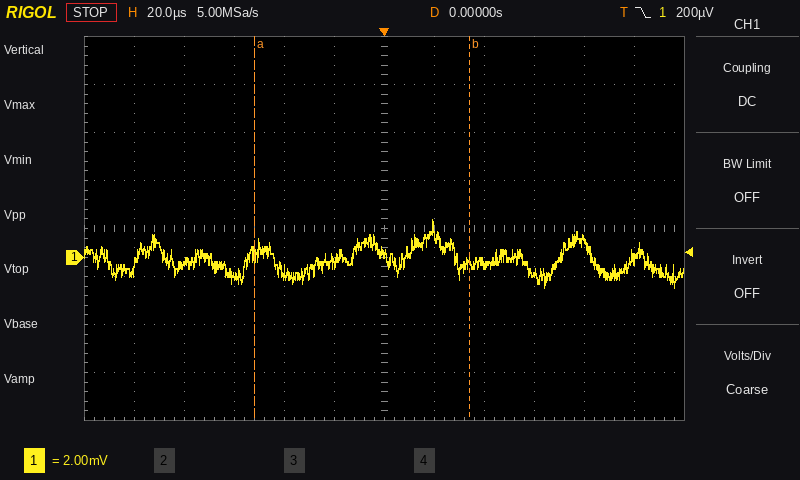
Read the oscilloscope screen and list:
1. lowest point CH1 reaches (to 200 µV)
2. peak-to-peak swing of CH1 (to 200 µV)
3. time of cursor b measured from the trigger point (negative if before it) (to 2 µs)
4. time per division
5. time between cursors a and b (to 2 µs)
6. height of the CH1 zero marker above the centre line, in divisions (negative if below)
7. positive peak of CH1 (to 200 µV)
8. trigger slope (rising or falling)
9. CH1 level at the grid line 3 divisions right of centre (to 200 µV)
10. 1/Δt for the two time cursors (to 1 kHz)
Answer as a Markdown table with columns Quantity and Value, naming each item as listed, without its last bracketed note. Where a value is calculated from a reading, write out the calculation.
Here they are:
| Quantity | Value |
|---|---|
| lowest point CH1 reaches | -1.2 mV |
| peak-to-peak swing of CH1 | 1.6 mV − (-1.2 mV) = 2.8 mV |
| time of cursor b measured from the trigger point (negative if before it) | +34 µs |
| time per division | 20 µs |
| time between cursors a and b | 86 µs |
| height of the CH1 zero marker above the centre line, in divisions | -0.6 div |
| positive peak of CH1 | 1.6 mV |
| trigger slope | falling |
| CH1 level at the grid line 3 divisions right of centre | -600 µV |
| 1/Δt for the two time cursors | 1 / 86 µs ≈ 12 kHz |
